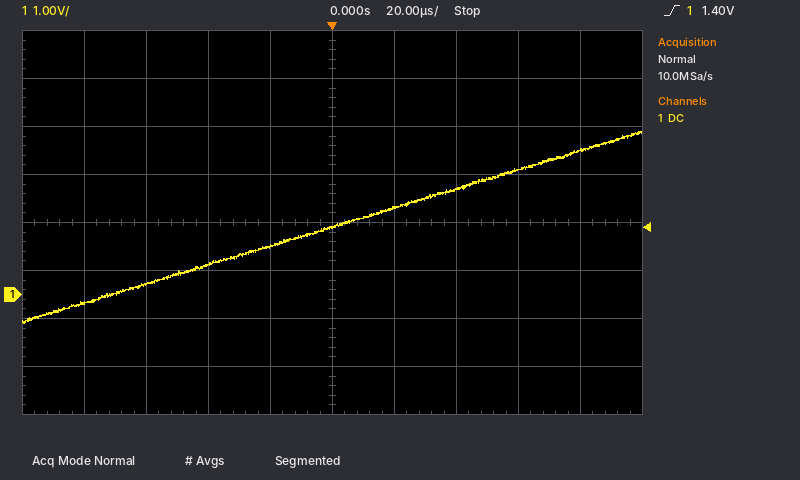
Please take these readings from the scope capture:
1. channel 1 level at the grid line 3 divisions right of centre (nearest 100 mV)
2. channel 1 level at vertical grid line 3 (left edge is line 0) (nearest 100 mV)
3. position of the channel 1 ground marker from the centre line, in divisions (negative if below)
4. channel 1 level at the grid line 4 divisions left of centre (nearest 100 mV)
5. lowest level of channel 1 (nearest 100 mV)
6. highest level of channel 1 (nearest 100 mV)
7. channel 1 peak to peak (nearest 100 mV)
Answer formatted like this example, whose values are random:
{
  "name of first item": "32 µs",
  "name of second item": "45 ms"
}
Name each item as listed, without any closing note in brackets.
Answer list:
{
  "channel 1 level at the grid line 3 divisions right of centre": "2.6 V",
  "channel 1 level at vertical grid line 3 (left edge is line 0)": "600 mV",
  "position of the channel 1 ground marker from the centre line, in divisions": "-1.5 div",
  "channel 1 level at the grid line 4 divisions left of centre": "-200 mV",
  "lowest level of channel 1": "-600 mV",
  "highest level of channel 1": "3.4 V",
  "channel 1 peak to peak": "4.0 V"
}
